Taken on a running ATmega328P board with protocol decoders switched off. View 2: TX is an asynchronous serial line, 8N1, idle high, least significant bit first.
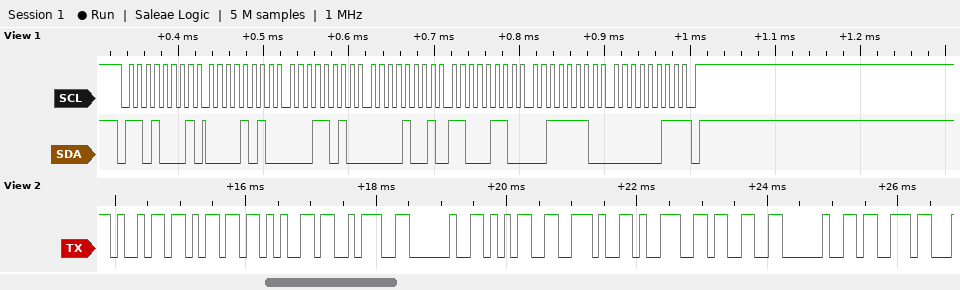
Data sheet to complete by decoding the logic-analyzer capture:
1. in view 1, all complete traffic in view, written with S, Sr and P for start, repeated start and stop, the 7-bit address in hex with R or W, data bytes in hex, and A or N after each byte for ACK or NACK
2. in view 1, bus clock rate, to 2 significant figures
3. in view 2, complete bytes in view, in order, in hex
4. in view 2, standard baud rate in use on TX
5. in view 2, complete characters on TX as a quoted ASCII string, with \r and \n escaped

S 68R A 0A A 1A A 09 A C6 A 3E A 03 N P
100 kHz
69 6D 65 3A 20 35 2E 39 33 20 73
9600 baud
"ime: 5.93 s"
